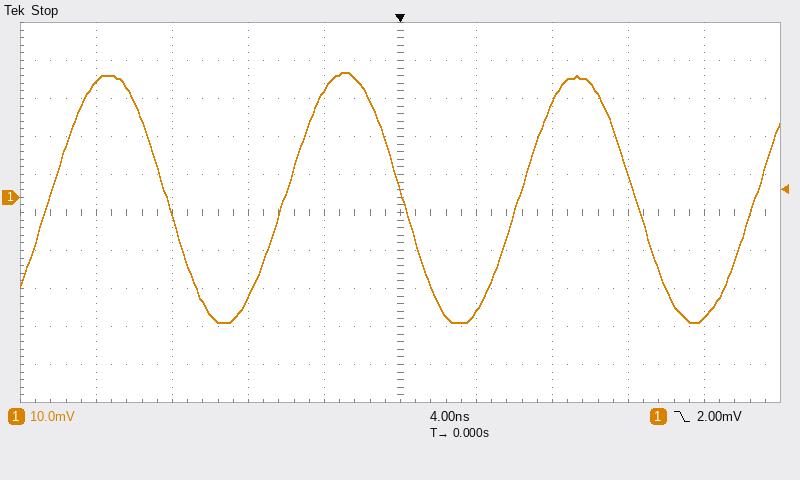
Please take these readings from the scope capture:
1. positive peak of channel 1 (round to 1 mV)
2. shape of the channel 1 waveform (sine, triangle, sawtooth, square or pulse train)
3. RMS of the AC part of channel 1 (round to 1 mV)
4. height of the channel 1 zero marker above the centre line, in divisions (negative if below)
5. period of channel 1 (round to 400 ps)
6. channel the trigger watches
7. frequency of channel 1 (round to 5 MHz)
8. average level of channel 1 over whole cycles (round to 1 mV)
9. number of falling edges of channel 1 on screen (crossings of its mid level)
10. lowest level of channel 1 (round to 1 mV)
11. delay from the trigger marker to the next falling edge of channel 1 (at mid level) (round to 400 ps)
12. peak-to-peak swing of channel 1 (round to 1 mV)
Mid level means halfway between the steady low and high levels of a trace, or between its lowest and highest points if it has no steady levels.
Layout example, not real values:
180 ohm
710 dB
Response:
33 mV
sine
23 mV
+0.4 div
12.4 ns
channel 1
80 MHz
0 mV
3
-33 mV
12.4 ns
66 mV
